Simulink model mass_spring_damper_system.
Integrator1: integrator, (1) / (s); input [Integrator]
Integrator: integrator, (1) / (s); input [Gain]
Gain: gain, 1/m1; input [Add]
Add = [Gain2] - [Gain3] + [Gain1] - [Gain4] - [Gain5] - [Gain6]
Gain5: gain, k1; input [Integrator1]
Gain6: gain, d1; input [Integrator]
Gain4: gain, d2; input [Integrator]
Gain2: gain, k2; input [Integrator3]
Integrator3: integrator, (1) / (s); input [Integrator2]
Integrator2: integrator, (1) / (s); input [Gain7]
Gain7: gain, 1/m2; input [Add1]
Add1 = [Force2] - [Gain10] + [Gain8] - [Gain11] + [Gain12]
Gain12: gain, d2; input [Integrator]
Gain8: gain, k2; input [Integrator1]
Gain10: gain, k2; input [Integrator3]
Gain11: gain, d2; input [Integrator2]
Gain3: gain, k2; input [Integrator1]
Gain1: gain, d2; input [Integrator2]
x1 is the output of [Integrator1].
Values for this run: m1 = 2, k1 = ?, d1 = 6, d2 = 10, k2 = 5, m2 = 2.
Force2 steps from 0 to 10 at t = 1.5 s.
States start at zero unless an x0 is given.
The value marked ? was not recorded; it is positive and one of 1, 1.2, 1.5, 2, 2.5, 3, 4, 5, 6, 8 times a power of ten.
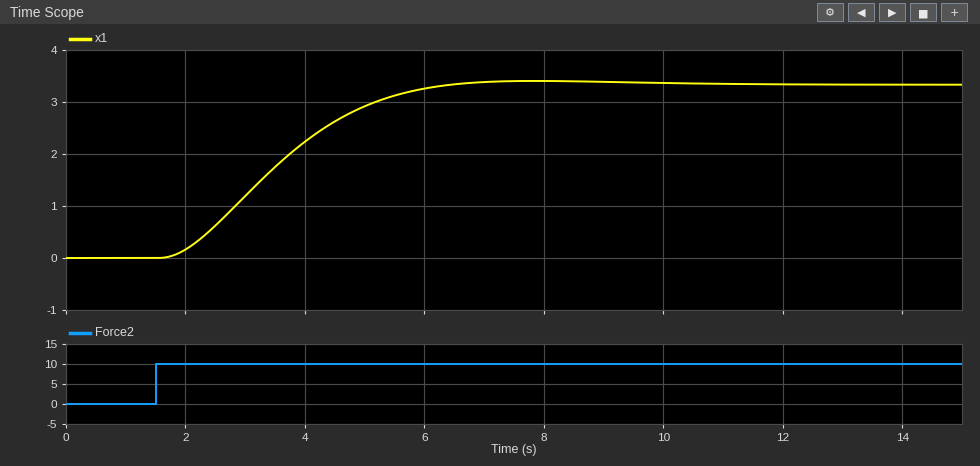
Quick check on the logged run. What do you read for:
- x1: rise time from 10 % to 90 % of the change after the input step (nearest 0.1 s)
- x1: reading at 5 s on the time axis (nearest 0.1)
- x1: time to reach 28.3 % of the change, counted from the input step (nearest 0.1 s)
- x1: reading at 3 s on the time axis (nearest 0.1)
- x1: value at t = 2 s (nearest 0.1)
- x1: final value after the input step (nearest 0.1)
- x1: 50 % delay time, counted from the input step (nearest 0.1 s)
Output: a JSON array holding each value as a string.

["3.0 s", "2.9", "1.3 s", "1.2", "0.2", "3.3", "1.9 s"]
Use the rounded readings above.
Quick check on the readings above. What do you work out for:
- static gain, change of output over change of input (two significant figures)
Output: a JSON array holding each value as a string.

["0.33"]
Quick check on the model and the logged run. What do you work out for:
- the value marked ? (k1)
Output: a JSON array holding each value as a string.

["3"]
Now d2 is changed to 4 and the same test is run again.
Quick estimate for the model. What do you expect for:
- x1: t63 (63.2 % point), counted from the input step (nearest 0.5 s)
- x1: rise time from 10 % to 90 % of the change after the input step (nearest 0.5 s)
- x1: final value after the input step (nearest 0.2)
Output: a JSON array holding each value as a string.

["2.5 s", "2.5 s", "3.4"]
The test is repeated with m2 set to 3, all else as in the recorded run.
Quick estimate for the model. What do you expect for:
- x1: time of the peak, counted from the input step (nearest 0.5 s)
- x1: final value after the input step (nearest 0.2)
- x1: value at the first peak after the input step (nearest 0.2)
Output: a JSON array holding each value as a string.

["6.0 s", "3.4", "3.6"]
